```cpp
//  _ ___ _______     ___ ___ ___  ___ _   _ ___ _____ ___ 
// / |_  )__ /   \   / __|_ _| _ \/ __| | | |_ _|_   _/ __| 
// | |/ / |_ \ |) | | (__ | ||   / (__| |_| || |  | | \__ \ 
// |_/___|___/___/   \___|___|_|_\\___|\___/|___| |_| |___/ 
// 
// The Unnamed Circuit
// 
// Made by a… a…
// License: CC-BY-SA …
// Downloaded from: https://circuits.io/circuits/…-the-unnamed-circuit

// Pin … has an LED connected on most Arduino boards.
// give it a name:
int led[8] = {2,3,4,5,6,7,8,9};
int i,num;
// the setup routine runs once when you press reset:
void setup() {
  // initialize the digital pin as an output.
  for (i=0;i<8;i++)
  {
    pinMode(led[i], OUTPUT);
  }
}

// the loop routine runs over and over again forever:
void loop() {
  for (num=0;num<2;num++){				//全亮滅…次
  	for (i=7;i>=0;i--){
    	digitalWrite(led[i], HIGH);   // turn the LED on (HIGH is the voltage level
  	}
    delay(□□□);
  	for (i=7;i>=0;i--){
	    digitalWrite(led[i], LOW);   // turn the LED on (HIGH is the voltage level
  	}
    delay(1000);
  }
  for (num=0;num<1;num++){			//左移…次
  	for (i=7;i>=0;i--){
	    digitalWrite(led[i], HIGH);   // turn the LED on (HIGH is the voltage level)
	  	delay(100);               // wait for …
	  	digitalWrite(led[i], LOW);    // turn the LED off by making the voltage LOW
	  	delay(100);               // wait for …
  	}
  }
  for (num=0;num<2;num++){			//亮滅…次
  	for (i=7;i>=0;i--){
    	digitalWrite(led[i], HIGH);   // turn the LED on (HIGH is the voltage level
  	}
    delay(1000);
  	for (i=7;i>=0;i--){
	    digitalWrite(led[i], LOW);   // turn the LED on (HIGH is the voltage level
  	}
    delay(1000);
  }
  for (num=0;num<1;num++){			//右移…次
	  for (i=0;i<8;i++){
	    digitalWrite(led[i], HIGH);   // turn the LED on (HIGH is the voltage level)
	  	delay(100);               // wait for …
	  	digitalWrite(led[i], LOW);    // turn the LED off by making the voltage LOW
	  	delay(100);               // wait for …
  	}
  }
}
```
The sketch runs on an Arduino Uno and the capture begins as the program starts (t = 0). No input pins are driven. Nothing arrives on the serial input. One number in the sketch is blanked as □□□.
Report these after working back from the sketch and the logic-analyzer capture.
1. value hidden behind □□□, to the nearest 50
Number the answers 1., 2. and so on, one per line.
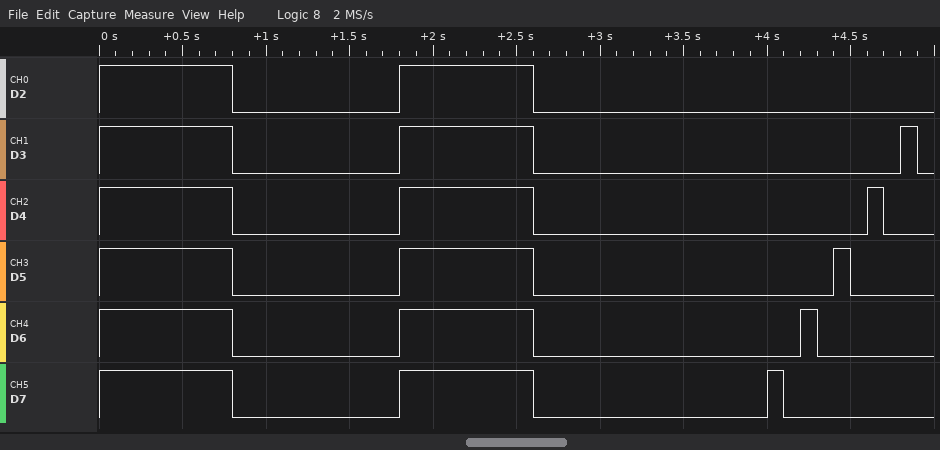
1. 800
